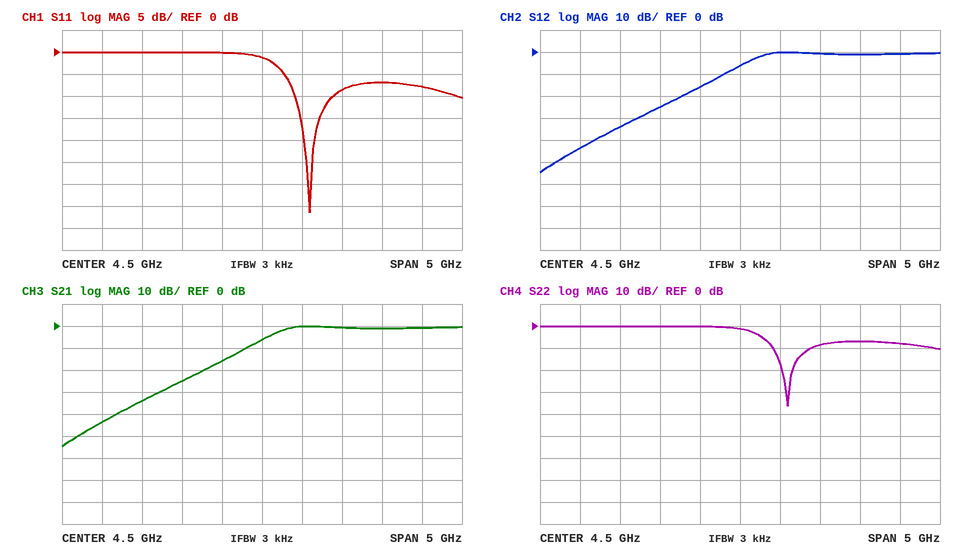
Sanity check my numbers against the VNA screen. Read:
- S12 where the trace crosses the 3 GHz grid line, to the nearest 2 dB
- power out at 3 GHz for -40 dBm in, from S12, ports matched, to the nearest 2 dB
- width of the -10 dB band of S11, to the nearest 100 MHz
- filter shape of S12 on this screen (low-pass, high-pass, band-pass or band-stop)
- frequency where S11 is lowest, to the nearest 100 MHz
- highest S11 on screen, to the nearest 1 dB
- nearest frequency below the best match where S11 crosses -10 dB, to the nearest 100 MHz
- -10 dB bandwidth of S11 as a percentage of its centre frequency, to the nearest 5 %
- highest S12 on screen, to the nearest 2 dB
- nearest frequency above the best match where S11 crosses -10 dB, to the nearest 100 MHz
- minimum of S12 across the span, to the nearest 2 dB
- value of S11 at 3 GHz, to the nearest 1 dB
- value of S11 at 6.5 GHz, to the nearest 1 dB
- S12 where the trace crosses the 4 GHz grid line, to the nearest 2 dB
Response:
-34 dB
-74 dBm
500 MHz
high-pass
5.1 GHz
0 dB
4.9 GHz
10 %
0 dB
5.4 GHz
-54 dB
0 dB
-8 dB
-16 dB
